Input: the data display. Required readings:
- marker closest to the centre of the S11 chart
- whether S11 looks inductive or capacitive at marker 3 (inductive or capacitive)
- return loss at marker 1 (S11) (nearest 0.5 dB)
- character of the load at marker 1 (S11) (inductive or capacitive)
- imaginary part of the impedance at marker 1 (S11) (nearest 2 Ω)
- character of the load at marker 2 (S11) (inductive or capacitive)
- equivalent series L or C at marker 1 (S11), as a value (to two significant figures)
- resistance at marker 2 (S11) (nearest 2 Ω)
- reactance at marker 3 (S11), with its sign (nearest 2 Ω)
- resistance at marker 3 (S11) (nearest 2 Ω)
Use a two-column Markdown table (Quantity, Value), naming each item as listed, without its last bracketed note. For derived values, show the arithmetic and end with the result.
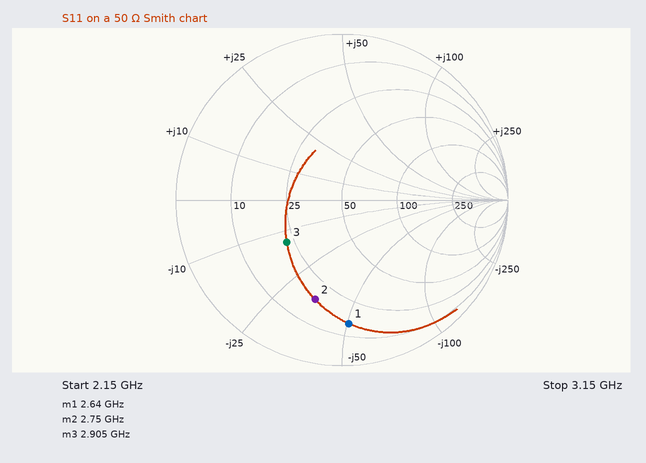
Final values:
| Quantity | Value |
|---|---|
| marker closest to the centre of the S11 chart | marker 3 |
| whether S11 looks inductive or capacitive at marker 3 | capacitive |
| return loss at marker 1 (S11) | 2.5 dB |
| character of the load at marker 1 (S11) | capacitive |
| imaginary part of the impedance at marker 1 (S11) | -50 Ω |
| character of the load at marker 2 (S11) | capacitive |
| equivalent series L or C at marker 1 (S11), as a value | C = 1/(2π × 2.64 GHz × 50 Ω) ≈ 1.2 pF |
| resistance at marker 2 (S11) | 18 Ω |
| reactance at marker 3 (S11), with its sign | -14 Ω |
| resistance at marker 3 (S11) | 22 Ω |
